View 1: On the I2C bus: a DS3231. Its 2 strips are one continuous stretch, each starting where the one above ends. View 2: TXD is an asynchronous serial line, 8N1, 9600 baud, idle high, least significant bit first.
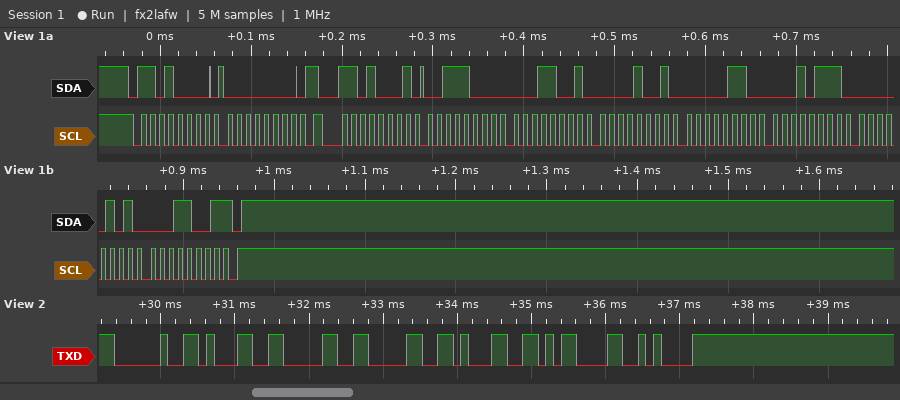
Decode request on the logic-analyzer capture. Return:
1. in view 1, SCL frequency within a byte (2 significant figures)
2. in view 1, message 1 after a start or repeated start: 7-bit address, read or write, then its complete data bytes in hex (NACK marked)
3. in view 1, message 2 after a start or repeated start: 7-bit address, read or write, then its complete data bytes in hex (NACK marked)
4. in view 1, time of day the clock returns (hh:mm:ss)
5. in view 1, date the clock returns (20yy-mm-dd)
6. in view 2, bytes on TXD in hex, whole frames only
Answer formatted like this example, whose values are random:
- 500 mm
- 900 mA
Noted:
- 100 kHz
- 0x68 write: 00
- 0x68 read: 38 19 09 06 17 05 19 NACK
- 09:19:38
- 2019-05-17
- 20 31 30 30 31 0D 0A
